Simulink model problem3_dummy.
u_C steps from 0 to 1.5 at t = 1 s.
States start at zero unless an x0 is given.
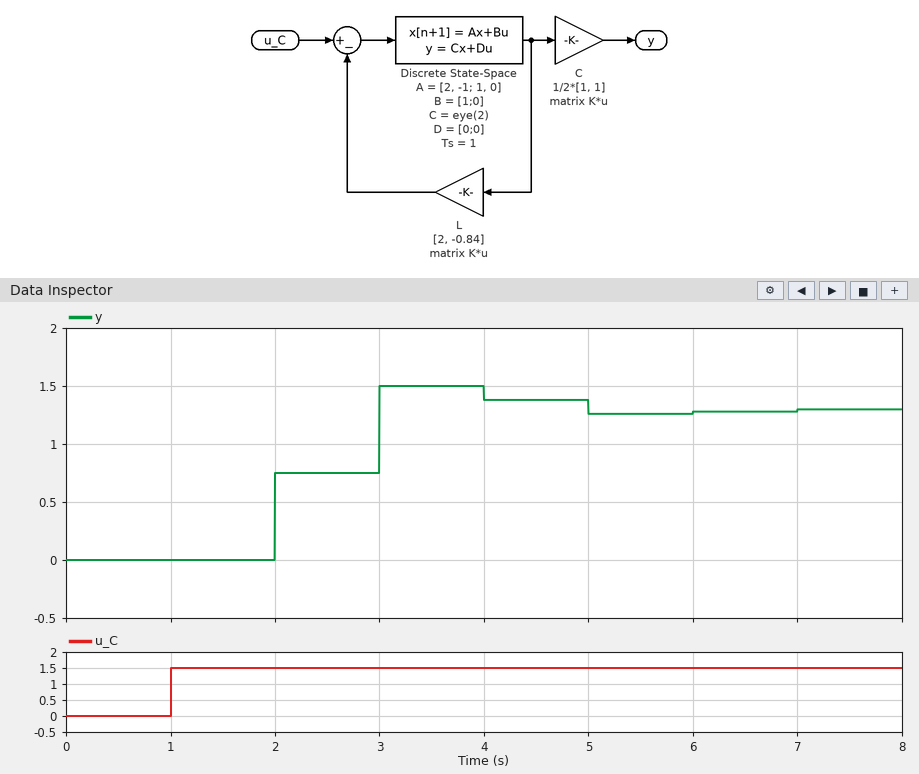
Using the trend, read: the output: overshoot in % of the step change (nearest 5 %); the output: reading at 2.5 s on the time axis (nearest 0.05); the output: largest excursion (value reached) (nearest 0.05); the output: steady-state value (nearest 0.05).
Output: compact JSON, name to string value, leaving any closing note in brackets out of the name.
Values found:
{"the output: overshoot in % of the step change": "15 %", "the output: reading at 2.5 s on the time axis": "0.75", "the output: largest excursion (value reached)": "1.50", "the output: steady-state value": "1.30"}
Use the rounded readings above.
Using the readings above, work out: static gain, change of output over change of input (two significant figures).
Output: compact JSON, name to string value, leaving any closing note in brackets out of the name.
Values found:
{"static gain, change of output over change of input": "0.87"}
